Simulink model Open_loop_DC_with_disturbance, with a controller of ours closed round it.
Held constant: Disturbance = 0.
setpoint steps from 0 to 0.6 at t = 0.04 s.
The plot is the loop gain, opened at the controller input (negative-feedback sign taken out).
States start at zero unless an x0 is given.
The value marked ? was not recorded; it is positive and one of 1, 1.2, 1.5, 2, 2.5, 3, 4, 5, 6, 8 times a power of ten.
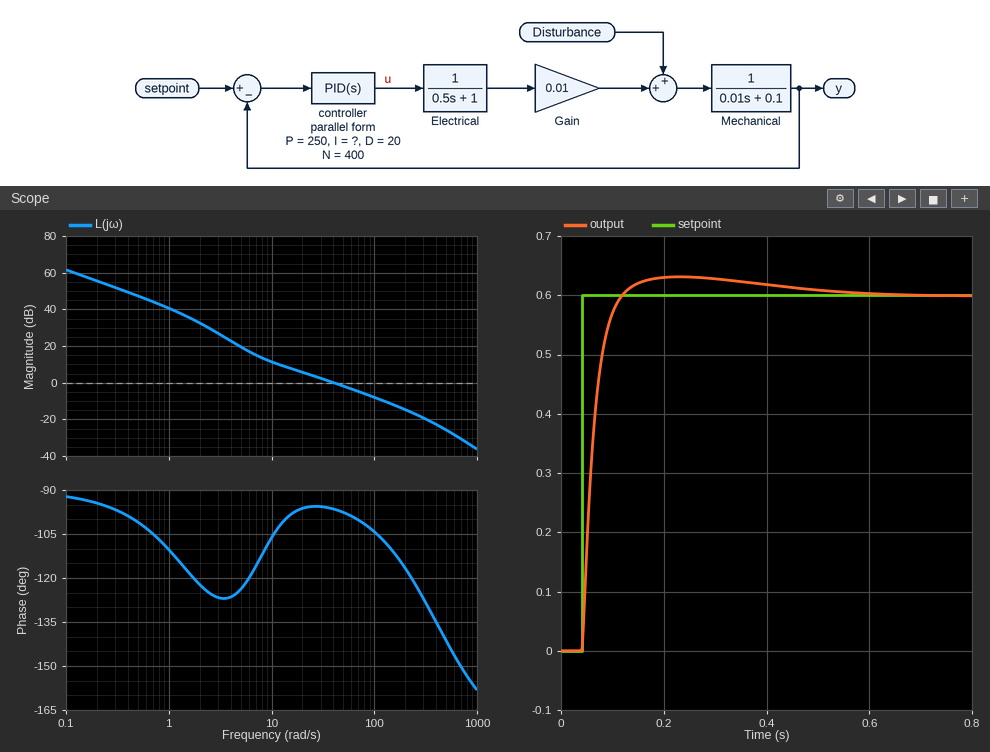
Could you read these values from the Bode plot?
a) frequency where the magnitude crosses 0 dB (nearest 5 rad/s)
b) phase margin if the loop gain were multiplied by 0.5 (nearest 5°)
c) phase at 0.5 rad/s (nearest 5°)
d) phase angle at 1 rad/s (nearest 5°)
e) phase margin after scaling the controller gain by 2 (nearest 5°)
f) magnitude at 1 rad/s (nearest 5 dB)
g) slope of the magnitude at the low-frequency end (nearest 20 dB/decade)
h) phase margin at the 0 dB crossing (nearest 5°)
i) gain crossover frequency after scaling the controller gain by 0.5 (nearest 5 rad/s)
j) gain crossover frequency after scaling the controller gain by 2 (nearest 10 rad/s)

40 rad/s
85°
-100°
-110°
80°
40 dB
-20 dB/decade
85°
20 rad/s
80 rad/s
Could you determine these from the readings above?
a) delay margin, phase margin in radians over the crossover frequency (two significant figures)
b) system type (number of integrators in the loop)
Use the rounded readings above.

0.037 s
1
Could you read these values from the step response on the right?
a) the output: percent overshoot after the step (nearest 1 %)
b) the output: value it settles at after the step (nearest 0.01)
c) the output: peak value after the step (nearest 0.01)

5 %
0.60
0.63
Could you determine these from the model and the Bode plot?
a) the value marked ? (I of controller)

1200
